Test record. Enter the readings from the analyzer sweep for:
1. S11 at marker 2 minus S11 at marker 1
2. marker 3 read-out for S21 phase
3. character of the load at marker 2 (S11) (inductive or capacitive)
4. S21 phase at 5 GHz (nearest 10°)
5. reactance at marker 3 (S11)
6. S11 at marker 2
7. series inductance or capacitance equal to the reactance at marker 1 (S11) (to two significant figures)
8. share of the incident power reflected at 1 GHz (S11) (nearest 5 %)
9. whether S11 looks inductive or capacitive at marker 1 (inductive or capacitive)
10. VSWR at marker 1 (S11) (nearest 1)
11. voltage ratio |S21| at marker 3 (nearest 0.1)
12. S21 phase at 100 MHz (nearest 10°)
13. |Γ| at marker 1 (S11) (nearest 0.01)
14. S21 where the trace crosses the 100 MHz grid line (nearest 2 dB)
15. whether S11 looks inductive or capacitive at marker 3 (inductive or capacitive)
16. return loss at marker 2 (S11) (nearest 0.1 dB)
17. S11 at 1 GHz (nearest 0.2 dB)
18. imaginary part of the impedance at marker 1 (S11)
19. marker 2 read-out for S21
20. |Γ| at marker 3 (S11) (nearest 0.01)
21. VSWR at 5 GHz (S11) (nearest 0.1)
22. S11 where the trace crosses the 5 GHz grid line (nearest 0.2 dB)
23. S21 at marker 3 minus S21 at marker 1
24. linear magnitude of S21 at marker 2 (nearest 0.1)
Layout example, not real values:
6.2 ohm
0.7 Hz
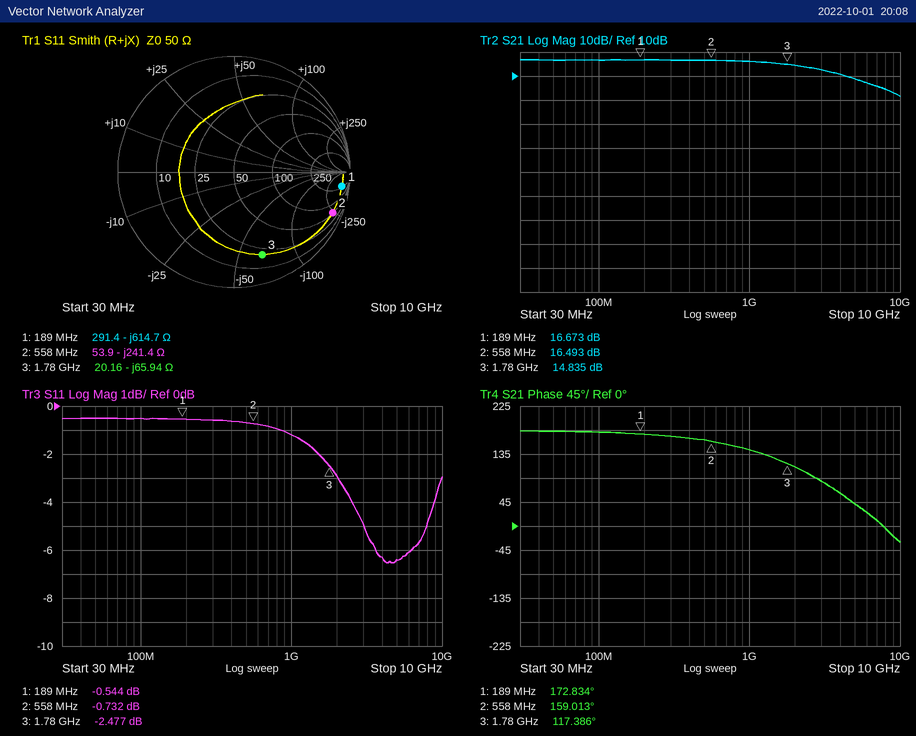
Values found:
-0.188 dB
117.386°
capacitive
40°
-65.94 Ω
-0.732 dB
1.4 pF
75 %
capacitive
32
5.5
180°
0.94
16 dB
capacitive
0.7 dB
-1.2 dB
-614.7 Ω
16.493 dB
0.75
2.8
-6.4 dB
-1.838 dB
6.7
